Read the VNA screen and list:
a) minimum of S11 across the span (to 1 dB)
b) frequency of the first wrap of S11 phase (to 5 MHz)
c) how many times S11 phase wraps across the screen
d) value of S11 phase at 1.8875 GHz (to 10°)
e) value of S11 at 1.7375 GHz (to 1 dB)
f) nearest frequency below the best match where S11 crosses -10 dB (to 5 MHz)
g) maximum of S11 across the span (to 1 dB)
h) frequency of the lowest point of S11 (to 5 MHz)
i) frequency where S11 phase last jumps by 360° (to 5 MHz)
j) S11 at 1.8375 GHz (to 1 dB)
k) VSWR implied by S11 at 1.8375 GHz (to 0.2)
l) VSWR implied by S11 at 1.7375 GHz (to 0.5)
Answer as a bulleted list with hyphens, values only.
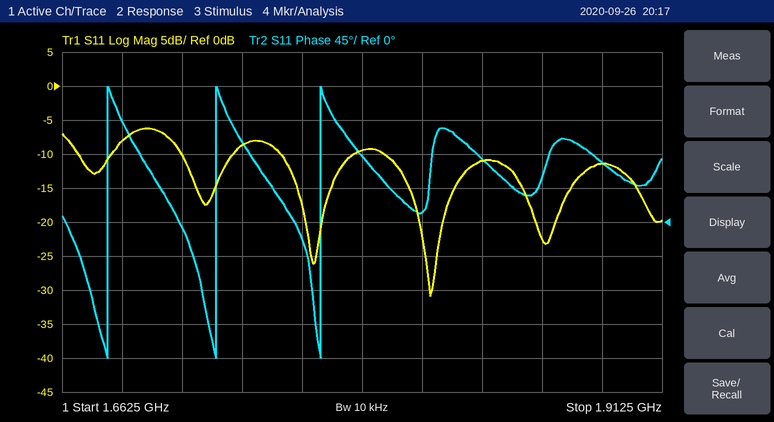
- -31 dB
- 1.680 GHz
- 3
- 80°
- -9 dB
- 1.795 GHz
- -6 dB
- 1.815 GHz
- 1.770 GHz
- -11 dB
- 1.8
- 2.0
